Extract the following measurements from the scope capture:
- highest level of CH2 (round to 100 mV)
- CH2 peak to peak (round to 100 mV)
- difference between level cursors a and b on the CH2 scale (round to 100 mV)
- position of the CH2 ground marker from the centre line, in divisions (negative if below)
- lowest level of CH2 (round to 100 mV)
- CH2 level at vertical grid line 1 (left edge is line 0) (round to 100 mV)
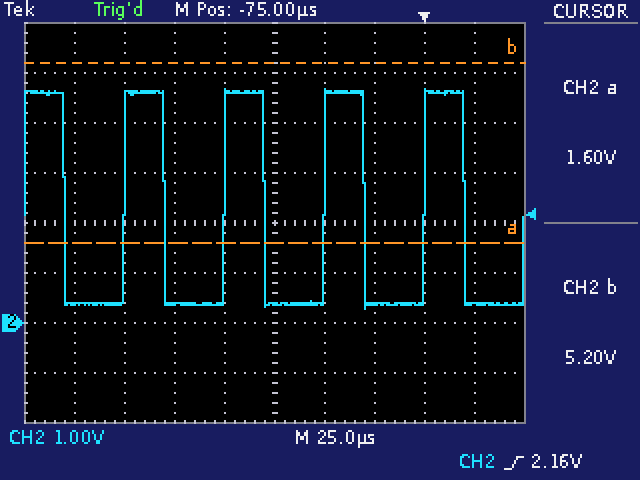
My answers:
4.7 V
4.4 V
3.6 V
-2.0 div
300 mV
400 mV
